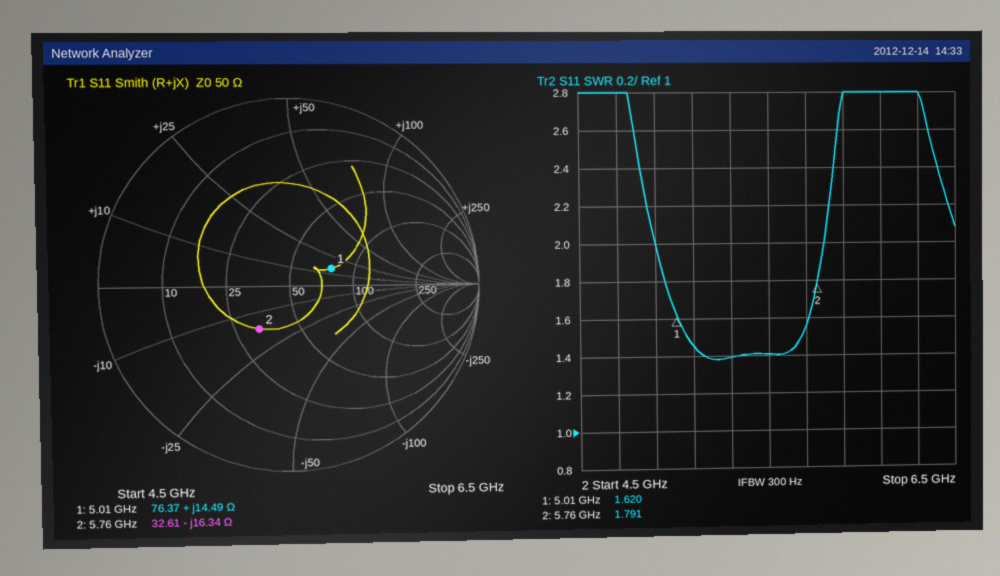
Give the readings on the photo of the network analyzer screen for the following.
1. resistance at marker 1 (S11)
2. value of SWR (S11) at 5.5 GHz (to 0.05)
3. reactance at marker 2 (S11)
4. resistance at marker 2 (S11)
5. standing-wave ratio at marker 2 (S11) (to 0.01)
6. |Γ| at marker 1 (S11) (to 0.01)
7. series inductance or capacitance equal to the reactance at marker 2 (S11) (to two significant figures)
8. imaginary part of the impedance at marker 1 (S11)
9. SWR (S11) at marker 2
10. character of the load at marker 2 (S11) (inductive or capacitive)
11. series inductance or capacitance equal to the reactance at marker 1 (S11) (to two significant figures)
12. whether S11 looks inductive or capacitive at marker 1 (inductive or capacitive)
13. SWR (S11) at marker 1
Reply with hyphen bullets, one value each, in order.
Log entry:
- 76.37 Ω
- 1.40
- -16.34 Ω
- 32.61 Ω
- 1.79
- 0.24
- 1.7 pF
- +14.49 Ω
- 1.791
- capacitive
- 460 pH
- inductive
- 1.620
